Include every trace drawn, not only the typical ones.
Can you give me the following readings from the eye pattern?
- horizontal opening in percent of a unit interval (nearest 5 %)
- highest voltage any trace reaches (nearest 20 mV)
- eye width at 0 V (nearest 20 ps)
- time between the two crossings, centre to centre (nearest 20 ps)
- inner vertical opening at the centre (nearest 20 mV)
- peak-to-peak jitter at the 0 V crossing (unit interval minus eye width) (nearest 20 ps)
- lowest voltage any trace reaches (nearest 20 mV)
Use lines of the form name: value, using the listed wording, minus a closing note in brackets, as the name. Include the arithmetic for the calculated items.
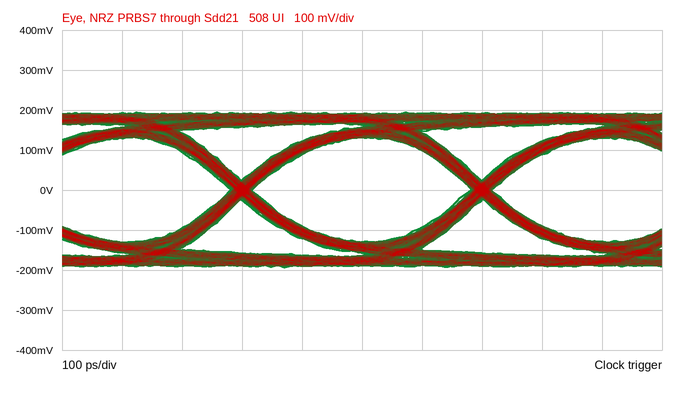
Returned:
horizontal opening in percent of a unit interval: 360 ps / 400 ps ≈ 90 %
highest voltage any trace reaches: 200 mV
eye width at 0 V: 360 ps
time between the two crossings, centre to centre: 400 ps
inner vertical opening at the centre: 260 mV
peak-to-peak jitter at the 0 V crossing (unit interval minus eye width): 40 ps
lowest voltage any trace reaches: -200 mV
